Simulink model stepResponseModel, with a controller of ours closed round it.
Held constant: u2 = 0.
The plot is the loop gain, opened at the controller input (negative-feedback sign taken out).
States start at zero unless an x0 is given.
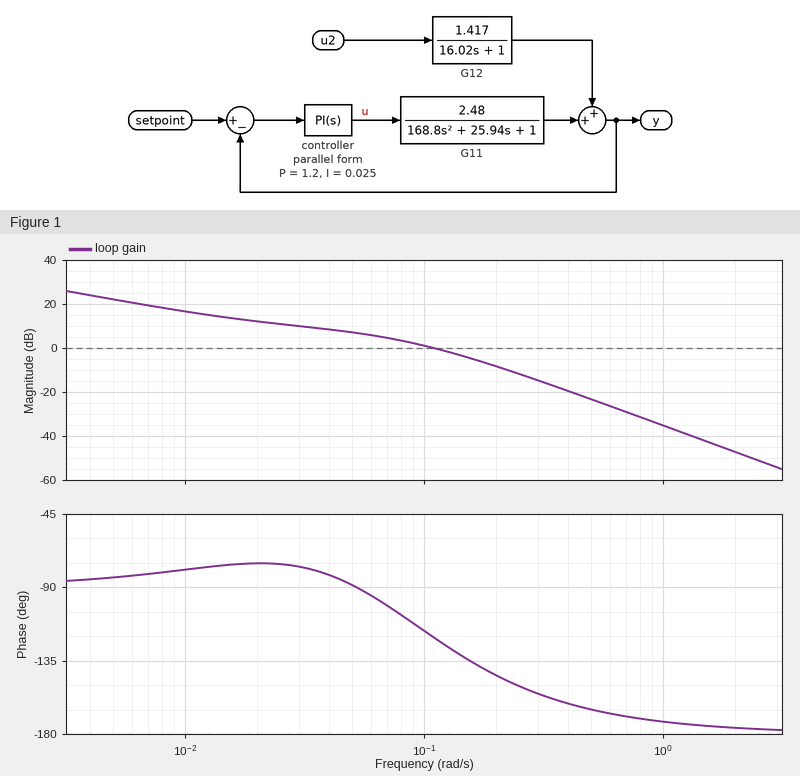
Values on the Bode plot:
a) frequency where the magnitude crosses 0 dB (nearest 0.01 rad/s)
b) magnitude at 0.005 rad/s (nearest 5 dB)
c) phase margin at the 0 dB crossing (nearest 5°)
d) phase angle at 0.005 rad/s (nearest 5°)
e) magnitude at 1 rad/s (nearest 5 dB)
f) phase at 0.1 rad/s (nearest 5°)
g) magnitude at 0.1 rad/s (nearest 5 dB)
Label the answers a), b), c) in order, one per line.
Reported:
a) 0.11 rad/s
b) 20 dB
c) 60°
d) -85°
e) -35 dB
f) -115°
g) 0 dB
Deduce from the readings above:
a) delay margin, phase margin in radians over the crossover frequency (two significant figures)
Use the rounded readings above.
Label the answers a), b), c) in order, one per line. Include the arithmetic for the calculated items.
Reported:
a) 60 × π / 180 / 0.11 = 9.5 s
